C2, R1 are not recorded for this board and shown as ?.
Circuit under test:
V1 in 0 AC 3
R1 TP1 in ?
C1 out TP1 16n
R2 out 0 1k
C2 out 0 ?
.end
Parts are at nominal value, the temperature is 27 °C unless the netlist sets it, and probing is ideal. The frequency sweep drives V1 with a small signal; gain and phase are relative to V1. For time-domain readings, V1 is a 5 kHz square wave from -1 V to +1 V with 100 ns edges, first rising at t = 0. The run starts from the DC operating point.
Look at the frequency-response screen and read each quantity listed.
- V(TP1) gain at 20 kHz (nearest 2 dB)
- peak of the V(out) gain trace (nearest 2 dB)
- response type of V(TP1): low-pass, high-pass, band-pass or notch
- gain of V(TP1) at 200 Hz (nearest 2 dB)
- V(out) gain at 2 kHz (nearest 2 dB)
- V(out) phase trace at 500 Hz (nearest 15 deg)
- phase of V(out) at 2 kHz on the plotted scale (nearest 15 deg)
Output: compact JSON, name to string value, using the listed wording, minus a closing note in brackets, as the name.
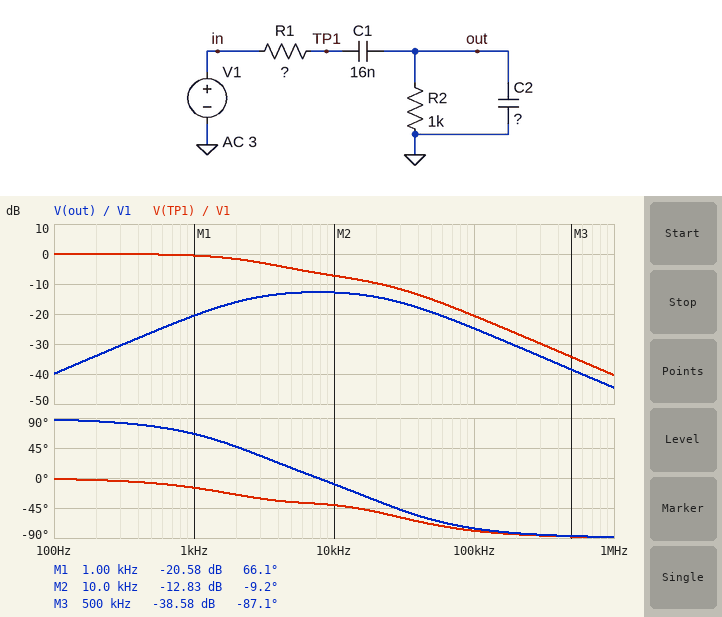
{"V(TP1) gain at 20 kHz": "-10 dB", "peak of the V(out) gain trace": "-12 dB", "response type of V(TP1): low-pass, high-pass, band-pass or notch": "low-pass", "gain of V(TP1) at 200 Hz": "0 dB", "V(out) gain at 2 kHz": "-16 dB", "V(out) phase trace at 500 Hz": "75 deg", "phase of V(out) at 2 kHz on the plotted scale": "45 deg"}
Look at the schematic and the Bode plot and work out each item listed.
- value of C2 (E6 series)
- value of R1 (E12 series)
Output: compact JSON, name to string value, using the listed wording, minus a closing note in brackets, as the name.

{"value of C2": "10 nF", "value of R1": "2.7 kΩ"}
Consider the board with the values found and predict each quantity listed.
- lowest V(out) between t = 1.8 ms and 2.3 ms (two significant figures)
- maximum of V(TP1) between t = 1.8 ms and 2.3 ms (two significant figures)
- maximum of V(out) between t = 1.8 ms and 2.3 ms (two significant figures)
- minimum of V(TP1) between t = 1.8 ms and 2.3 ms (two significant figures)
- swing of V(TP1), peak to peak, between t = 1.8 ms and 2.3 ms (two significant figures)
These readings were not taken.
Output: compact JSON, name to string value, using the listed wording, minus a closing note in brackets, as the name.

{"lowest V(out) between t = 1.8 ms and 2.3 ms": "-320 mV", "maximum of V(TP1) between t = 1.8 ms and 2.3 ms": "780 mV", "maximum of V(out) between t = 1.8 ms and 2.3 ms": "320 mV", "minimum of V(TP1) between t = 1.8 ms and 2.3 ms": "-780 mV", "swing of V(TP1), peak to peak, between t = 1.8 ms and 2.3 ms": "1.6 V"}
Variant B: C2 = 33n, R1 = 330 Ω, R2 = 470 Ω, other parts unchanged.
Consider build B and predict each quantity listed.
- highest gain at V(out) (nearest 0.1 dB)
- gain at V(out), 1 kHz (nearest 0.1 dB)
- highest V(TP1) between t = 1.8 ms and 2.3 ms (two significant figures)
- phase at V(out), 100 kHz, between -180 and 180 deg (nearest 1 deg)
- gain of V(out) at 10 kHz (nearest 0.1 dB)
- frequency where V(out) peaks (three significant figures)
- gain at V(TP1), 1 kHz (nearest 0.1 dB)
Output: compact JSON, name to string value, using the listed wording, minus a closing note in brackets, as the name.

{"highest gain at V(out)": "-11.5 dB", "gain at V(out), 1 kHz": "-26.6 dB", "highest V(TP1) between t = 1.8 ms and 2.3 ms": "1.0 V", "phase at V(out), 100 kHz, between -180 and 180 deg": "-60 deg", "gain of V(out) at 10 kHz": "-12.1 dB", "frequency where V(out) peaks": "17.6 kHz", "gain at V(TP1), 1 kHz": "0 dB"}
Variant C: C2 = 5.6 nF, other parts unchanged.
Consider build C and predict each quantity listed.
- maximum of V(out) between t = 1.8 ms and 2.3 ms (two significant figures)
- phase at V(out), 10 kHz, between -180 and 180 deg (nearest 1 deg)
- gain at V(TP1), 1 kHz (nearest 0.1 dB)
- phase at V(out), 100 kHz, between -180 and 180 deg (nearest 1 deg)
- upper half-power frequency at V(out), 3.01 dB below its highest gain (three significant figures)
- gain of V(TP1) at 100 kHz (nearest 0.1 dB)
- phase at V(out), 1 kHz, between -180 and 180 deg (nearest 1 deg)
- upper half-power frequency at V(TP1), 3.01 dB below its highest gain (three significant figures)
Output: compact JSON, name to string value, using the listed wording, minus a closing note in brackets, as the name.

{"maximum of V(out) between t = 1.8 ms and 2.3 ms": "360 mV", "phase at V(out), 10 kHz, between -180 and 180 deg": "1 deg", "gain at V(TP1), 1 kHz": "-0.5 dB", "phase at V(out), 100 kHz, between -180 and 180 deg": "-67 deg", "upper half-power frequency at V(out), 3.01 dB below its highest gain": "45.0 kHz", "gain of V(TP1) at 100 kHz": "-17.6 dB", "phase at V(out), 1 kHz, between -180 and 180 deg": "68 deg", "upper half-power frequency at V(TP1), 3.01 dB below its highest gain": "3.01 kHz"}
